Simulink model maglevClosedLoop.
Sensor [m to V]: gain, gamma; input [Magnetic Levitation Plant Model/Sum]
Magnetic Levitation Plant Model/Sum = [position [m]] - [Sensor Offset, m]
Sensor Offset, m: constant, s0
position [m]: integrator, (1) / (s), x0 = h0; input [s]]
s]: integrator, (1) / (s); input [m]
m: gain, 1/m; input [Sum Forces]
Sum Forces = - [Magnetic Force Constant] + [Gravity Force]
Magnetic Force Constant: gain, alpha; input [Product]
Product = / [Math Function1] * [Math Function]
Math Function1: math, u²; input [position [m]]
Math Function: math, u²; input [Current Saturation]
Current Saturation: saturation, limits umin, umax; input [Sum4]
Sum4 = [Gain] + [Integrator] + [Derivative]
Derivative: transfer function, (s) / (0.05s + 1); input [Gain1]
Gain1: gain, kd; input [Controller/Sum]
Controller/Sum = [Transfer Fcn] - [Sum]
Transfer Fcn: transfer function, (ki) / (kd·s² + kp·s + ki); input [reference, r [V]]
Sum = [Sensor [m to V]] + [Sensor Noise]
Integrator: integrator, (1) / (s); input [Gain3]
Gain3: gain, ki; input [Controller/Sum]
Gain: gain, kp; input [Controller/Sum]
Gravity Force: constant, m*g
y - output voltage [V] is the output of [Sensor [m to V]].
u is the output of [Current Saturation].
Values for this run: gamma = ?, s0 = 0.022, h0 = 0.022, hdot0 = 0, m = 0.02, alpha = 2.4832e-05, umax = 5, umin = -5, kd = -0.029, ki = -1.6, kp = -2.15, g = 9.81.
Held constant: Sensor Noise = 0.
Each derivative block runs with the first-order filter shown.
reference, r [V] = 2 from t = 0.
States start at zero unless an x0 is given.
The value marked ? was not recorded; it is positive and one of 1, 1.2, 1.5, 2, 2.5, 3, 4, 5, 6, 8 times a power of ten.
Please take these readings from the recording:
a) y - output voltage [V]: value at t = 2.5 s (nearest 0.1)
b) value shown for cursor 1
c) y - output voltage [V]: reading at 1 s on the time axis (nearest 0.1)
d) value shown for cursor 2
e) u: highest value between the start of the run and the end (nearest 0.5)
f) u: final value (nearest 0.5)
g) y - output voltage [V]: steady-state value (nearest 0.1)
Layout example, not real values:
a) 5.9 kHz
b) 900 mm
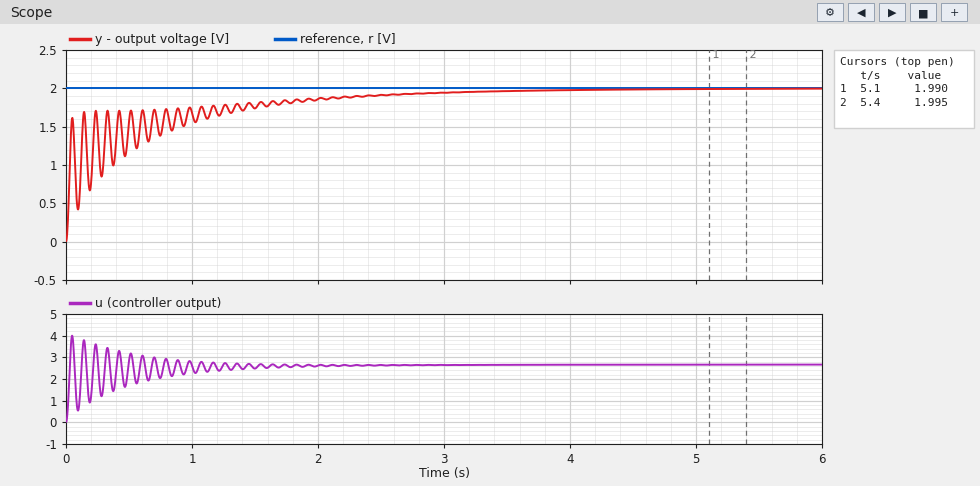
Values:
a) 1.9
b) 1.990
c) 1.7
d) 1.995
e) 4.0
f) 2.5
g) 2.0
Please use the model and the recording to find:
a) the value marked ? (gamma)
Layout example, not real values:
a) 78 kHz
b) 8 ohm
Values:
a) 250
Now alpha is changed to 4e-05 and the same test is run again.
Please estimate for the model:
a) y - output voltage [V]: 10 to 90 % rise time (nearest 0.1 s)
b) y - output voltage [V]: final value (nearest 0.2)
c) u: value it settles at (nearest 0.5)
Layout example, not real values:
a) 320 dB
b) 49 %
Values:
a) 2.0 s
b) 2.0
c) 2.0
